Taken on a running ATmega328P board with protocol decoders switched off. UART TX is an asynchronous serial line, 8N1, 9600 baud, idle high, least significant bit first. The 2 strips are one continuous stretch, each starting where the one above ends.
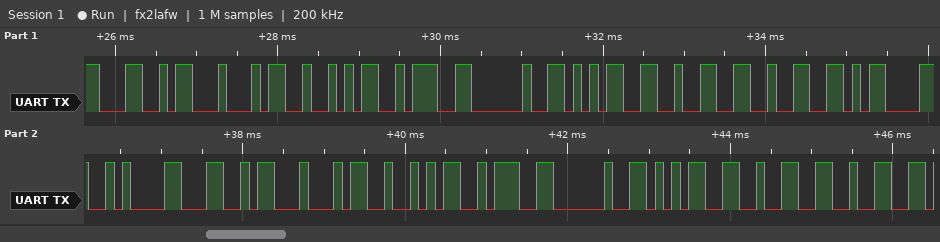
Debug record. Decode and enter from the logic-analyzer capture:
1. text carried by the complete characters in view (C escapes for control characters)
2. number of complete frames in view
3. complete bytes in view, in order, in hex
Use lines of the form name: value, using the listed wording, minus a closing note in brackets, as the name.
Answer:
text carried by the complete characters in view: "LDR: 522\r\nLDR: 522"
number of complete frames in view: 18
complete bytes in view, in order, in hex: 4C 44 52 3A 20 35 32 32 0D 0A 4C 44 52 3A 20 35 32 32
